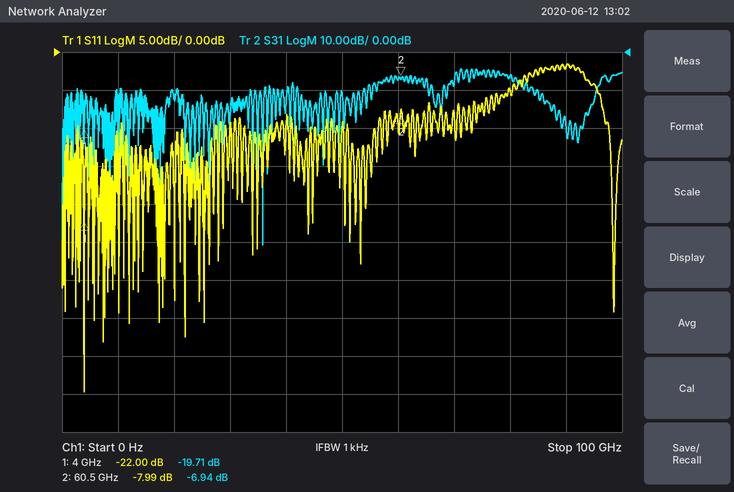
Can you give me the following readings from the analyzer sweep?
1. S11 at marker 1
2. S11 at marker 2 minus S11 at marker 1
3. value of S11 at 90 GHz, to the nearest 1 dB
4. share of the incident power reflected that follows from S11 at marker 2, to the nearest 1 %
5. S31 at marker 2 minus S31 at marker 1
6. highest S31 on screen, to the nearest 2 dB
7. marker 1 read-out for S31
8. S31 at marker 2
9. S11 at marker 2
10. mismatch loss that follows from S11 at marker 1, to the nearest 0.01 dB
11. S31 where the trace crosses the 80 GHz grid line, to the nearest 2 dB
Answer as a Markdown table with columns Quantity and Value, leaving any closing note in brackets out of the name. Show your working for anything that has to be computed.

| Quantity | Value |
|---|---|
| S11 at marker 1 | -22.00 dB |
| S11 at marker 2 minus S11 at marker 1 | -7.99 − (-22) = 14.01 dB |
| value of S11 at 90 GHz, to the nearest 1 dB | -2 dB |
| share of the incident power reflected that follows from S11 at marker 2, to the nearest 1 % | 10^(-7.99/10) ≈ 16 % |
| S31 at marker 2 minus S31 at marker 1 | -6.94 − (-19.71) = 12.77 dB |
| highest S31 on screen, to the nearest 2 dB | -4 dB |
| marker 1 read-out for S31 | -19.71 dB |
| S31 at marker 2 | -6.94 dB |
| S11 at marker 2 | -7.99 dB |
| mismatch loss that follows from S11 at marker 1, to the nearest 0.01 dB | −10 log10(1 − 10^(-22/10)) ≈ 0.03 dB |
| S31 where the trace crosses the 80 GHz grid line, to the nearest 2 dB | -6 dB |
